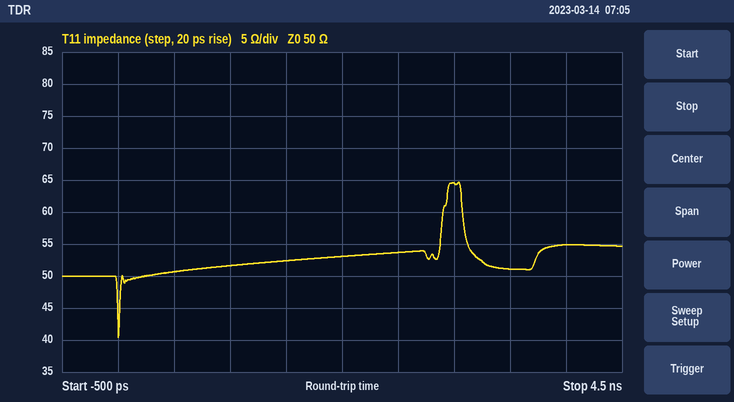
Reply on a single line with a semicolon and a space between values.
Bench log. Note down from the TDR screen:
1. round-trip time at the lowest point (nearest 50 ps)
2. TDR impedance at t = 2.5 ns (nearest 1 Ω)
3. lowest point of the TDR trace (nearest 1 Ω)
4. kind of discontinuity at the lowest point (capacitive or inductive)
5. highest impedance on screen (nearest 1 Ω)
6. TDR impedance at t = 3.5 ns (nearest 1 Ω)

0 ps; 54 Ω; 40 Ω; capacitive; 65 Ω; 51 Ω
